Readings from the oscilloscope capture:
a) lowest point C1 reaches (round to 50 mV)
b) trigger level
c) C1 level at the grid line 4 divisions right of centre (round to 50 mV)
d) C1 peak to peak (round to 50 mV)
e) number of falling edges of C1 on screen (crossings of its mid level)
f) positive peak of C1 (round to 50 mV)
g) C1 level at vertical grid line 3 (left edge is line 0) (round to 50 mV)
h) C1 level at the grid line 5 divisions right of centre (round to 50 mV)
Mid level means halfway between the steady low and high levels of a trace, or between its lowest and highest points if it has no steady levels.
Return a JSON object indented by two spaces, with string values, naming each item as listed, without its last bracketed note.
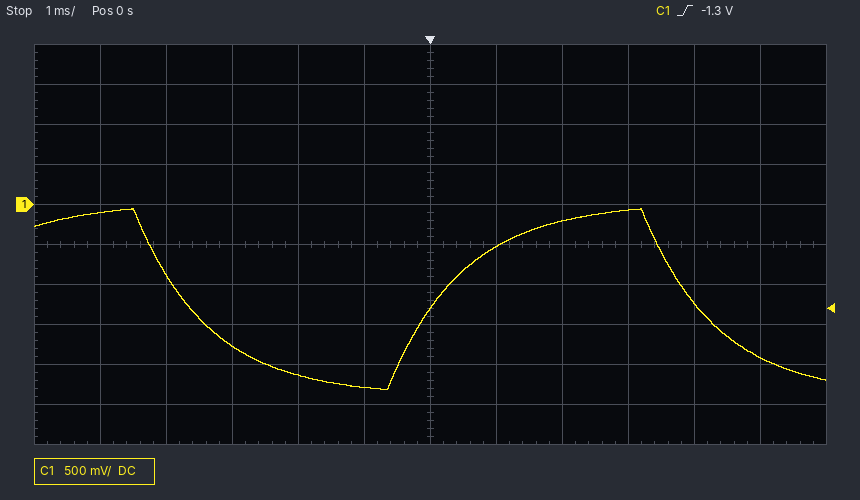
{
  "lowest point C1 reaches": "-2.30 V",
  "trigger level": "-1.3 V",
  "C1 level at the grid line 4 divisions right of centre": "-1.25 V",
  "C1 peak to peak": "2.25 V",
  "number of falling edges of C1 on screen": "2",
  "positive peak of C1": "-50 mV",
  "C1 level at vertical grid line 3 (left edge is line 0)": "-1.75 V",
  "C1 level at the grid line 5 divisions right of centre": "-1.90 V"
}
